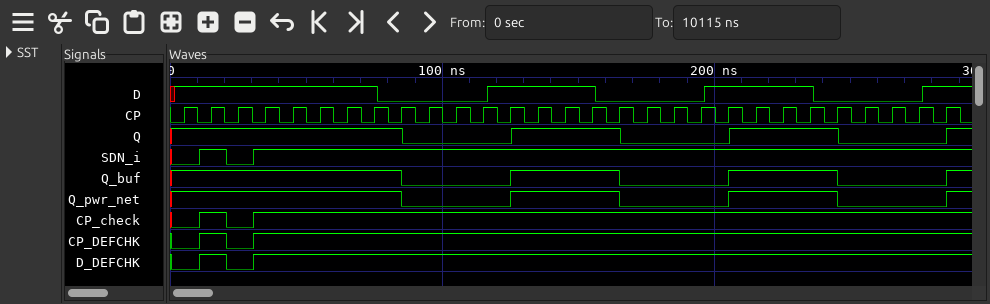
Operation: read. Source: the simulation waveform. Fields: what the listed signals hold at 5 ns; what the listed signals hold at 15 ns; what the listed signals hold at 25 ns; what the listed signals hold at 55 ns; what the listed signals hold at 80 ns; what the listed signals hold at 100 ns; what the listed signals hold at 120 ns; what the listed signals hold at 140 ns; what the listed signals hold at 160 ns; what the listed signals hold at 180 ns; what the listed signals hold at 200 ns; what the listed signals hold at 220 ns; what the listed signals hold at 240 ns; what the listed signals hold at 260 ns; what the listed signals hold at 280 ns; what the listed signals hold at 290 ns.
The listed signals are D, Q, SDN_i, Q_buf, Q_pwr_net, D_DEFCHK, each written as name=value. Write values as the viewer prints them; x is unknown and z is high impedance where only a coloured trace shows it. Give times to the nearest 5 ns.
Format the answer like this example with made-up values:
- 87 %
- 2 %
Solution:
- D=1, Q=1, SDN_i=0, Q_buf=1, Q_pwr_net=1, D_DEFCHK=0
- D=1, Q=1, SDN_i=1, Q_buf=1, Q_pwr_net=1, D_DEFCHK=1
- D=1, Q=1, SDN_i=0, Q_buf=1, Q_pwr_net=1, D_DEFCHK=0
- D=1, Q=1, SDN_i=1, Q_buf=1, Q_pwr_net=1, D_DEFCHK=1
- D=0, Q=1, SDN_i=1, Q_buf=1, Q_pwr_net=1, D_DEFCHK=1
- D=0, Q=0, SDN_i=1, Q_buf=0, Q_pwr_net=0, D_DEFCHK=1
- D=1, Q=0, SDN_i=1, Q_buf=0, Q_pwr_net=0, D_DEFCHK=1
- D=1, Q=1, SDN_i=1, Q_buf=1, Q_pwr_net=1, D_DEFCHK=1
- D=0, Q=1, SDN_i=1, Q_buf=1, Q_pwr_net=1, D_DEFCHK=1
- D=0, Q=0, SDN_i=1, Q_buf=0, Q_pwr_net=0, D_DEFCHK=1
- D=1, Q=0, SDN_i=1, Q_buf=0, Q_pwr_net=0, D_DEFCHK=1
- D=1, Q=1, SDN_i=1, Q_buf=1, Q_pwr_net=1, D_DEFCHK=1
- D=0, Q=1, SDN_i=1, Q_buf=1, Q_pwr_net=1, D_DEFCHK=1
- D=0, Q=0, SDN_i=1, Q_buf=0, Q_pwr_net=0, D_DEFCHK=1
- D=1, Q=0, SDN_i=1, Q_buf=0, Q_pwr_net=0, D_DEFCHK=1
- D=1, Q=1, SDN_i=1, Q_buf=1, Q_pwr_net=1, D_DEFCHK=1
